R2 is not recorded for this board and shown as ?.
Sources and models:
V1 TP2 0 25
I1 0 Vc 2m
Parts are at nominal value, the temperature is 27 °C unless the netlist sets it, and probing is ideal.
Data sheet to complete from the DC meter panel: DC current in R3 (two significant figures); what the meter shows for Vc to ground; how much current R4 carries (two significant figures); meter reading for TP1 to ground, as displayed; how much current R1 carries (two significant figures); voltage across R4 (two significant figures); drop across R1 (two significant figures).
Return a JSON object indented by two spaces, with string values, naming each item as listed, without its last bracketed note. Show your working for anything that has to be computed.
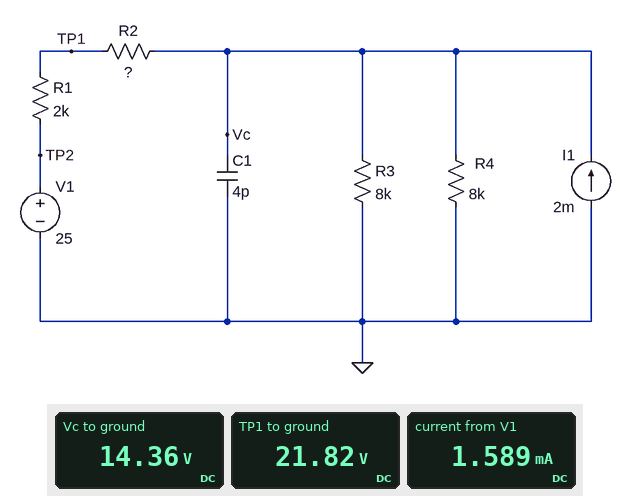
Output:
{
  "DC current in R3": "(14.36 V) / 8 kΩ = 1.8 mA",
  "what the meter shows for Vc to ground": "14.36 V",
  "how much current R4 carries": "(14.36 V) / 8 kΩ = 1.8 mA",
  "meter reading for TP1 to ground, as displayed": "21.82 V",
  "how much current R1 carries": "(25 V - 21.82 V) / 2 kΩ = 1.6 mA",
  "voltage across R4": "14.36 V = 14 V",
  "drop across R1": "25 V - 21.82 V = 3.2 V"
}
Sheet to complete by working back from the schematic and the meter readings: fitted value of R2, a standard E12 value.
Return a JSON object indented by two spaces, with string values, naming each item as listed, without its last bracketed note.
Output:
{
  "fitted value of R2, a standard E12 value": "4.7 kΩ"
}
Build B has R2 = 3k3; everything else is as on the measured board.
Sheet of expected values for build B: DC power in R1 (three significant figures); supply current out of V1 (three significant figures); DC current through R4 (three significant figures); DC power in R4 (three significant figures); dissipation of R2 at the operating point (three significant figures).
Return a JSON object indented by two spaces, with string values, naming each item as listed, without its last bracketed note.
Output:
{
  "DC power in R1": "6.68 mW",
  "supply current out of V1": "1.83 mA",
  "DC current through R4": "1.91 mA",
  "DC power in R4": "29.3 mW",
  "dissipation of R2 at the operating point": "11.0 mW"
}
